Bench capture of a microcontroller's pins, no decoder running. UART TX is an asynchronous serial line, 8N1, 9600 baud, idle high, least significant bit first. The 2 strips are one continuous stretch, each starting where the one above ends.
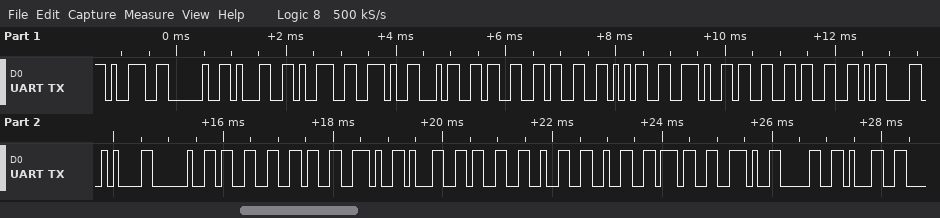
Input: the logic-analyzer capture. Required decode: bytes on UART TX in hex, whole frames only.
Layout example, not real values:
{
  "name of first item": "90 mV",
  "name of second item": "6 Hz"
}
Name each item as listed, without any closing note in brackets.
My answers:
{
  "bytes on UART TX in hex, whole frames only": "39 20 31 39 2E 34 33 33 35 2E 33 33 0D 0A 20 33 36 2E 31 33 32 32 37 2E 30 31"
}
